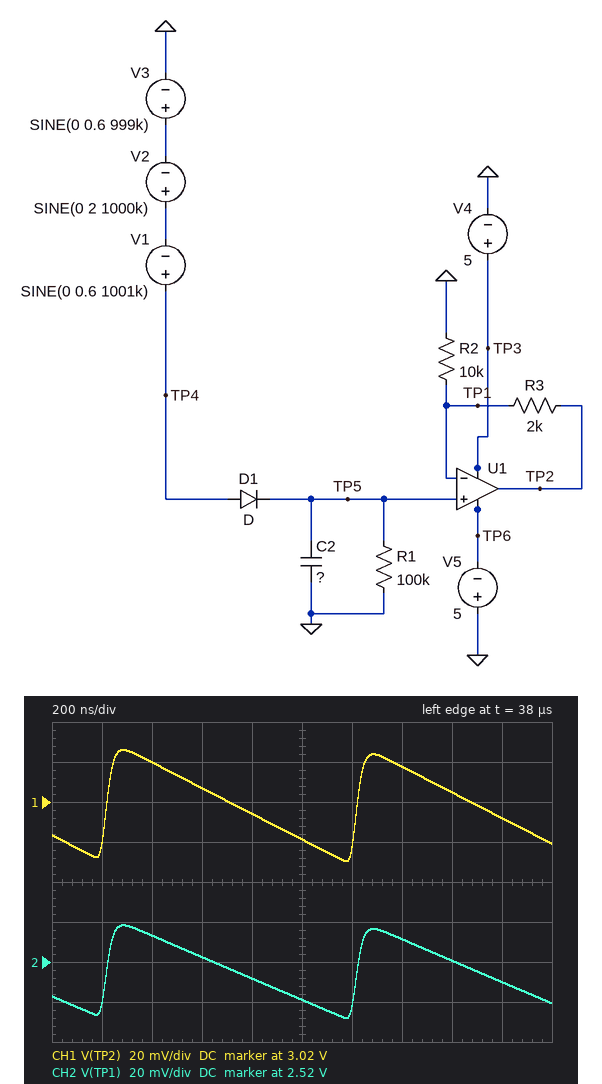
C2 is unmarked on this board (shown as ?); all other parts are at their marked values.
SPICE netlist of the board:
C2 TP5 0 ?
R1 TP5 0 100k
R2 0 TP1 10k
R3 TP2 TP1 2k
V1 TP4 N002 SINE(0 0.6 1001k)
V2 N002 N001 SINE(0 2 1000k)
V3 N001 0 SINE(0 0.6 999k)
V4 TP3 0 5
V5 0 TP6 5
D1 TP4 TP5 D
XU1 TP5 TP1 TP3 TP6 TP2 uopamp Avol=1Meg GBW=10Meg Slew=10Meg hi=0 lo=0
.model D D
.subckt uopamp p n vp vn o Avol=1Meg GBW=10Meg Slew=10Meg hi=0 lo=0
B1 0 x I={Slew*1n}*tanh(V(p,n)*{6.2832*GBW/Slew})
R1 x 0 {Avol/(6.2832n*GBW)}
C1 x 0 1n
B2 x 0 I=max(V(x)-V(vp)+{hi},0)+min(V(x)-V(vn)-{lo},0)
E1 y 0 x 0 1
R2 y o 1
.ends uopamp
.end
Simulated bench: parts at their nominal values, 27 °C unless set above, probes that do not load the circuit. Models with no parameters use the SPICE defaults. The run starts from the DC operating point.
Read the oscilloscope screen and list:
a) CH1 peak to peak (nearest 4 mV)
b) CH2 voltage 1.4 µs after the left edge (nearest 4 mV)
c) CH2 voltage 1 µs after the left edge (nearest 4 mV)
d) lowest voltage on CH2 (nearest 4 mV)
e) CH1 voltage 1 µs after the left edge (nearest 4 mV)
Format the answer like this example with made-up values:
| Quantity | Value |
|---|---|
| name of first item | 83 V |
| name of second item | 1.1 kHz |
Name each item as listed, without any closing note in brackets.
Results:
| Quantity | Value |
|---|---|
| CH1 peak to peak | 56 mV |
| CH2 voltage 1.4 µs after the left edge | 2.532 V |
| CH2 voltage 1 µs after the left edge | 2.500 V |
| lowest voltage on CH2 | 2.492 V |
| CH1 voltage 1 µs after the left edge | 3.000 V |
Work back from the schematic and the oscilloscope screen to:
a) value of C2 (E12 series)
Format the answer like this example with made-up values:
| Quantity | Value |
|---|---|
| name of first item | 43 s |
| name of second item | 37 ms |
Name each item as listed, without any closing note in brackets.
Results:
| Quantity | Value |
|---|---|
| value of C2 | 470 pF |
